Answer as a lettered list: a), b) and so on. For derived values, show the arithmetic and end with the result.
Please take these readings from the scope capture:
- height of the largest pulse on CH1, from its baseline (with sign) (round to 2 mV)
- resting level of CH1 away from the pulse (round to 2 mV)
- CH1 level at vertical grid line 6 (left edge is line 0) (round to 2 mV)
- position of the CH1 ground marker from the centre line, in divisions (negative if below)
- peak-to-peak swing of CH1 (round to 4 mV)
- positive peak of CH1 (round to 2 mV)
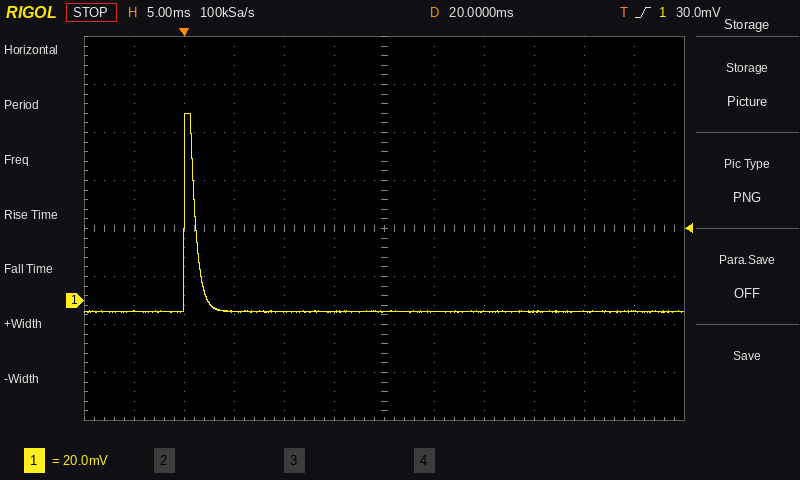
a) 78 mV − (-4 mV) = +82 mV
b) -4 mV
c) -4 mV
d) -1.5 div
e) 84 mV
f) 78 mV
